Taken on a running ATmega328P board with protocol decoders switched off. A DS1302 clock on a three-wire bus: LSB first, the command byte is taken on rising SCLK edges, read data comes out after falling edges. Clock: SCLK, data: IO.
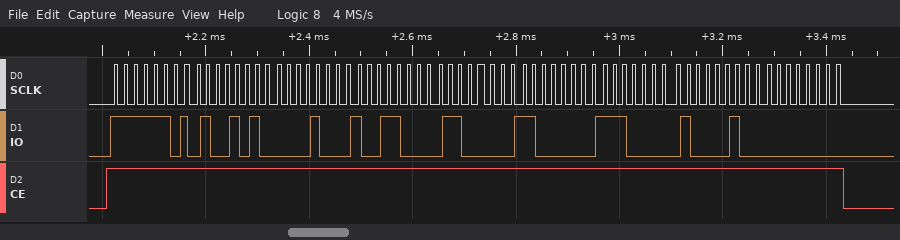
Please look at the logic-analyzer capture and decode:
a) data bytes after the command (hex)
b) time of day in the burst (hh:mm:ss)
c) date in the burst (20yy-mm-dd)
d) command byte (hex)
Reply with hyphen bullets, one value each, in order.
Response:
- 52 10 19 06 03 07 21 00
- 19:10:52
- 2021-03-06
- 0xBF
